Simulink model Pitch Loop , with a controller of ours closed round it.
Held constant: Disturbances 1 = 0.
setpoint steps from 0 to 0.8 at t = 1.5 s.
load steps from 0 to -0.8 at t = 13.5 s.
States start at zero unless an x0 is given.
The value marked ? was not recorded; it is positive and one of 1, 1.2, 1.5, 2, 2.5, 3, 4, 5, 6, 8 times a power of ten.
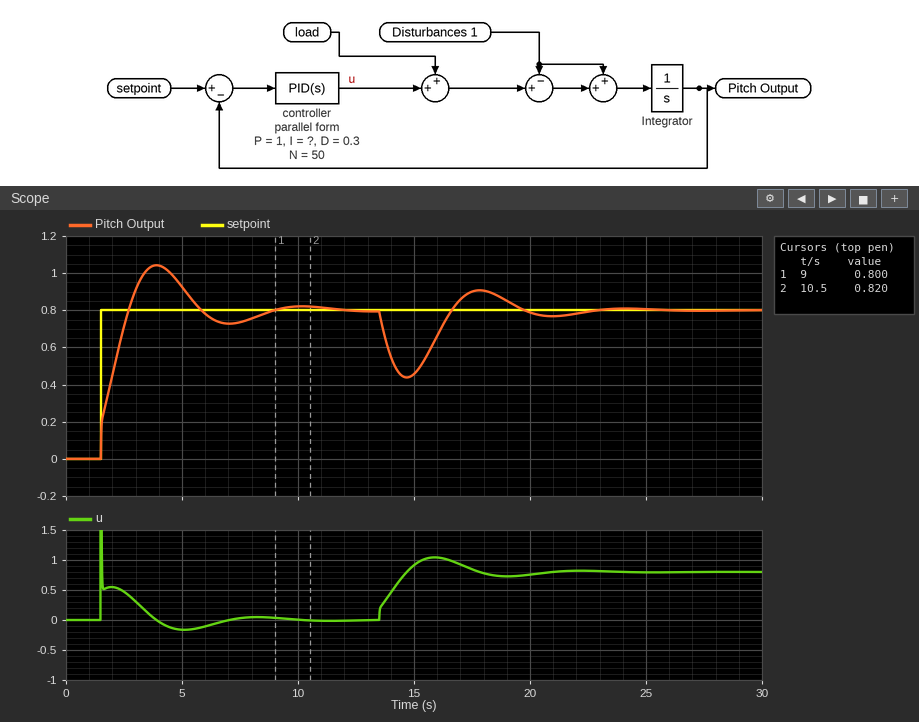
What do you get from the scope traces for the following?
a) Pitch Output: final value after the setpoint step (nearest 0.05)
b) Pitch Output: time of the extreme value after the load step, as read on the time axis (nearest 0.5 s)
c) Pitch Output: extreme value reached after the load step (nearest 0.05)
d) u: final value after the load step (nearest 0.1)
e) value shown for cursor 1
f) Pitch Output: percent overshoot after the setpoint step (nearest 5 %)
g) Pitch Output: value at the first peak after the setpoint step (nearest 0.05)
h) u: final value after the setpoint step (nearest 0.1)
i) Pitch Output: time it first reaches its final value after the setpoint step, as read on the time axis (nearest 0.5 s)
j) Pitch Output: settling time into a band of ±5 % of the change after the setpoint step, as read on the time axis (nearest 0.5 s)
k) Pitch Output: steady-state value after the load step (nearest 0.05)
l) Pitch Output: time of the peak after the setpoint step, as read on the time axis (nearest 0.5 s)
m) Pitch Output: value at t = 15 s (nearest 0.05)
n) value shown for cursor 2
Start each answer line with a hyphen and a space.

- 0.80
- 14.5 s
- 0.45
- 0.8
- 0.800
- 30 %
- 1.05
- 0.0
- 2.5 s
- 8.0 s
- 0.80
- 4.0 s
- 0.45
- 0.820
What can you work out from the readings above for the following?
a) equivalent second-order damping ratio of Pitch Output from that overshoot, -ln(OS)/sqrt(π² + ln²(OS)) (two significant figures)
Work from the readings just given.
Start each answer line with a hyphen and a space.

- 0.36
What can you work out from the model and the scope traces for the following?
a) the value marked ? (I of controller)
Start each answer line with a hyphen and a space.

- 1.5
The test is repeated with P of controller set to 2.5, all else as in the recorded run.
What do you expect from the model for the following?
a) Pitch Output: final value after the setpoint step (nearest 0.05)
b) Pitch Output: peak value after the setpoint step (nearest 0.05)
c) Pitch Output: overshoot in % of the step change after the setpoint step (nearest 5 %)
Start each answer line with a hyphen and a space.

- 0.80
- 0.90
- 10 %
